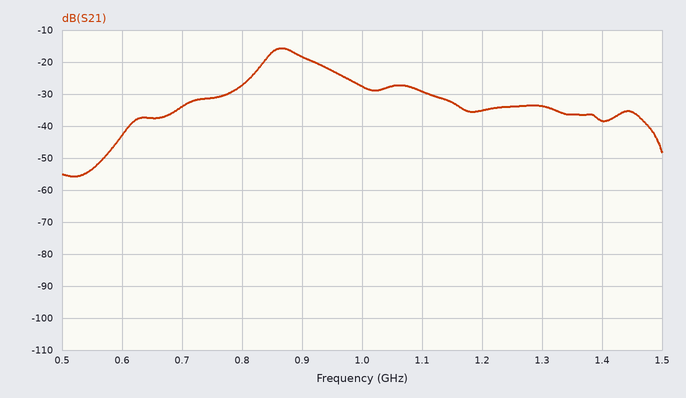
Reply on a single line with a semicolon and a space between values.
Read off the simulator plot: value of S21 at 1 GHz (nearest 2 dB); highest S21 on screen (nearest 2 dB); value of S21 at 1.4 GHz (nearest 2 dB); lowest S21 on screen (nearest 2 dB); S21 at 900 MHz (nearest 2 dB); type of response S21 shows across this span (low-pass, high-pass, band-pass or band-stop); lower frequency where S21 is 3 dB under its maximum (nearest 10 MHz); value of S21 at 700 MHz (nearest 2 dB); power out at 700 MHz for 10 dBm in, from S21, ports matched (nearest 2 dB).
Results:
-28 dB; -16 dB; -38 dB; -56 dB; -18 dB; band-pass; 840 MHz; -34 dB; -24 dBm
